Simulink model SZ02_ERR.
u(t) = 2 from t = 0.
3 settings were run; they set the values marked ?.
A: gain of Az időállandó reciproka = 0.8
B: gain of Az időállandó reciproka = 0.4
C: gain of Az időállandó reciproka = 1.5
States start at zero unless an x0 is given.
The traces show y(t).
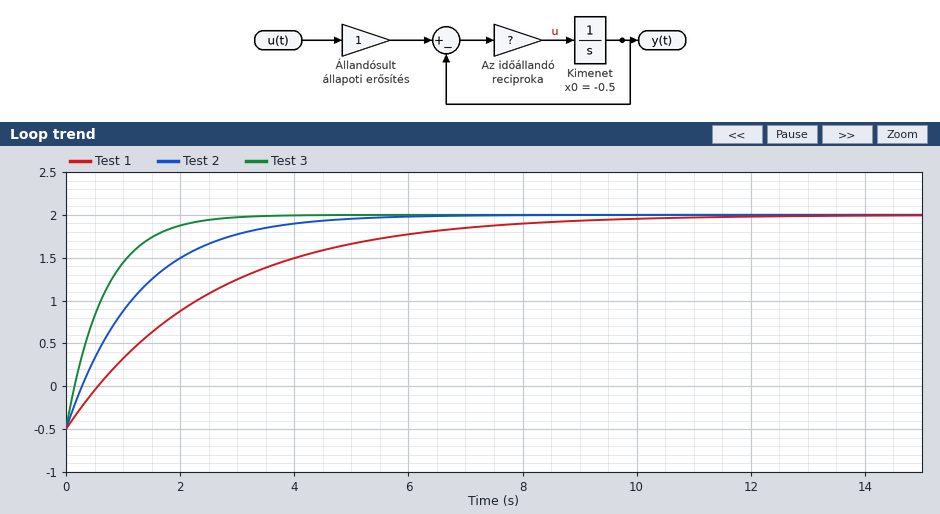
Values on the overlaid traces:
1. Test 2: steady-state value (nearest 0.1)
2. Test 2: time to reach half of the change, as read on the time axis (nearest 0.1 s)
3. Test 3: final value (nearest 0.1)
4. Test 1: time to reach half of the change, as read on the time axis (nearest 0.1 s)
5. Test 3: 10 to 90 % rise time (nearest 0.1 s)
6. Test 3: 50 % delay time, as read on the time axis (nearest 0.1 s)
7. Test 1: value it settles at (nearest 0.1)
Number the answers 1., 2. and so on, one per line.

1. 2.0
2. 0.9 s
3. 2.0
4. 1.7 s
5. 1.5 s
6. 0.5 s
7. 2.0
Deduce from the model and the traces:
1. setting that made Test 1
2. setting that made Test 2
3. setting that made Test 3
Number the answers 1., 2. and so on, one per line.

1. B
2. A
3. C
